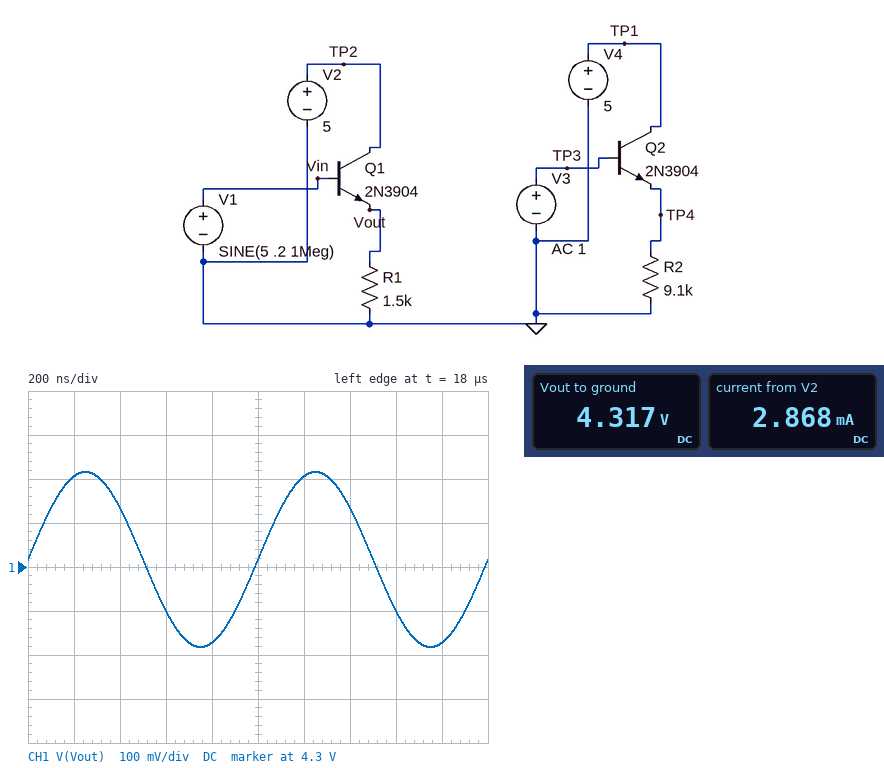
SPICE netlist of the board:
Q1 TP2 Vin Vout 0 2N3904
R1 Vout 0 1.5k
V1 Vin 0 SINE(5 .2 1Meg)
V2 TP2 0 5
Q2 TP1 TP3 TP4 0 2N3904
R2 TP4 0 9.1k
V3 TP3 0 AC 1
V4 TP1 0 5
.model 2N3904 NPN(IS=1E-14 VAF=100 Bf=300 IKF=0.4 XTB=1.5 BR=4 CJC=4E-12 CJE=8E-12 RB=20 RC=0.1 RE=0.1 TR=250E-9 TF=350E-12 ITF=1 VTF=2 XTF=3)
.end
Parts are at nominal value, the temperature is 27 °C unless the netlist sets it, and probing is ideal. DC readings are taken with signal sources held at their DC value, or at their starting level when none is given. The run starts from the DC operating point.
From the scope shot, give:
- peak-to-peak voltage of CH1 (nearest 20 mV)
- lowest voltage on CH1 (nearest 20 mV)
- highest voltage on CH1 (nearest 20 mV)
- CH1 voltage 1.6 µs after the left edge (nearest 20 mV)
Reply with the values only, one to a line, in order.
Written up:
400 mV
4.12 V
4.52 V
4.20 V
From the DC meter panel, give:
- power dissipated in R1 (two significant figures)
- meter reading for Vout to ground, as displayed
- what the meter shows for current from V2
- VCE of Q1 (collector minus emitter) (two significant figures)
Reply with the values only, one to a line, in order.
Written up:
12 mW
4.317 V
2.868 mA
680 mV
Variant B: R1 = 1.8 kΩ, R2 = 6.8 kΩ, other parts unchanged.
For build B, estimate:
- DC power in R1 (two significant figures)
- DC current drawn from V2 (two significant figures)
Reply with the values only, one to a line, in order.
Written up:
10 mW
2.4 mA
